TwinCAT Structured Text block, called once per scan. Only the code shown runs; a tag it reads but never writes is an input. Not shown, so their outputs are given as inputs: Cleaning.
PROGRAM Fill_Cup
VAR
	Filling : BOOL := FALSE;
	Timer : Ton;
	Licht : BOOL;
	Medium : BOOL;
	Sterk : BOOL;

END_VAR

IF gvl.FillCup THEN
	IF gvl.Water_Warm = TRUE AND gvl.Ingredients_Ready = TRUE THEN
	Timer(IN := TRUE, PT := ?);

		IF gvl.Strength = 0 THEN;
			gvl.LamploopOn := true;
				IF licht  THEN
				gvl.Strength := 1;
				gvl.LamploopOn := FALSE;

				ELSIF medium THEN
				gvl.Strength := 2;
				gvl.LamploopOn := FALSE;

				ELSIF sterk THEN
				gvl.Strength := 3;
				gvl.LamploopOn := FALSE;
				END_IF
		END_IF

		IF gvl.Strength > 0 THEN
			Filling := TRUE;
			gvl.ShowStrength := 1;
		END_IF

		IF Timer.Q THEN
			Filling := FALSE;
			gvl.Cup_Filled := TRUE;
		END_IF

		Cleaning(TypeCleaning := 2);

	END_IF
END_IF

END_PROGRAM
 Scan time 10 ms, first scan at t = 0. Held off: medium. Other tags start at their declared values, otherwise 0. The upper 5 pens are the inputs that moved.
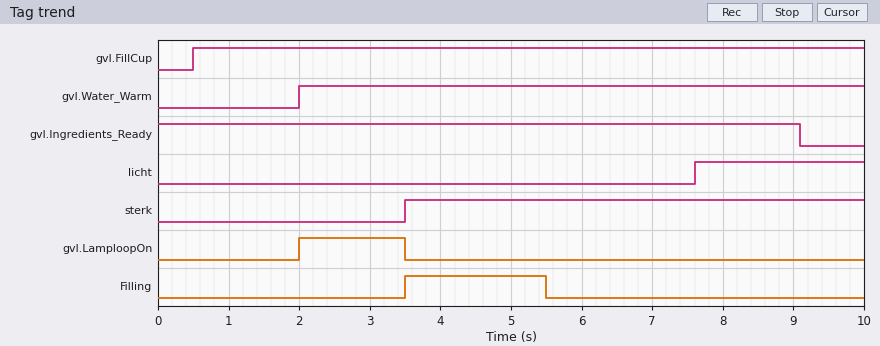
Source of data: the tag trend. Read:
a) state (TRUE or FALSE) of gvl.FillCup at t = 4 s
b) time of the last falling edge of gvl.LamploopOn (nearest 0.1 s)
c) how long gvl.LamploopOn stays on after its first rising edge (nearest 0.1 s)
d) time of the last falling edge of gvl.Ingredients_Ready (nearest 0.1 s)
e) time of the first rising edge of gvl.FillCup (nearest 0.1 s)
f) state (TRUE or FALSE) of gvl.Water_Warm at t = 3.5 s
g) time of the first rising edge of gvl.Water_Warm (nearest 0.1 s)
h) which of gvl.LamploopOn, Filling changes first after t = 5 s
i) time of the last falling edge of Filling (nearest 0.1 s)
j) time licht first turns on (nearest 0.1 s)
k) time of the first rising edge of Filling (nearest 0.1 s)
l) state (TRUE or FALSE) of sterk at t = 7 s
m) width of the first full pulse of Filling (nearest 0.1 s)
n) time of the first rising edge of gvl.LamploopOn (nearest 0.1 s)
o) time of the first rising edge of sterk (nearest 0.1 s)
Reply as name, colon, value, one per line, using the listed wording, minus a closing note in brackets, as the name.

state (TRUE or FALSE) of gvl.FillCup at t = 4 s: TRUE
time of the last falling edge of gvl.LamploopOn: 3.5 s
how long gvl.LamploopOn stays on after its first rising edge: 1.5 s
time of the last falling edge of gvl.Ingredients_Ready: 9.1 s
time of the first rising edge of gvl.FillCup: 0.5 s
state (TRUE or FALSE) of gvl.Water_Warm at t = 3.5 s: TRUE
time of the first rising edge of gvl.Water_Warm: 2.0 s
which of gvl.LamploopOn, Filling changes first after t = 5 s: Filling
time of the last falling edge of Filling: 5.5 s
time licht first turns on: 7.6 s
time of the first rising edge of Filling: 3.5 s
state (TRUE or FALSE) of sterk at t = 7 s: TRUE
width of the first full pulse of Filling: 2.0 s
time of the first rising edge of gvl.LamploopOn: 2.0 s
time of the first rising edge of sterk: 3.5 s
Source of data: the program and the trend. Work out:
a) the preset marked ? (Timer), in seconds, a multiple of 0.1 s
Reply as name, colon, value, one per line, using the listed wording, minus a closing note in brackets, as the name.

the preset marked ? (Timer), in seconds, a multiple of 0.1 s: 3.5 s
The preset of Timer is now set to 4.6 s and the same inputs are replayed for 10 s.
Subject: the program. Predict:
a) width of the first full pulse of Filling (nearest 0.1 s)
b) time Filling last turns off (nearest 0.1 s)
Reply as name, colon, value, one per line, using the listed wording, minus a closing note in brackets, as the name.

width of the first full pulse of Filling: 3.1 s
time Filling last turns off: 6.6 s
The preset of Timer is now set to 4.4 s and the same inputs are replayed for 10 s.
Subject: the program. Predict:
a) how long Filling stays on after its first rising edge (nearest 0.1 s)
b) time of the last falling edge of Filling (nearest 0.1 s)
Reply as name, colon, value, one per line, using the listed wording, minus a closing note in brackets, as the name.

how long Filling stays on after its first rising edge: 2.9 s
time of the last falling edge of Filling: 6.4 s
